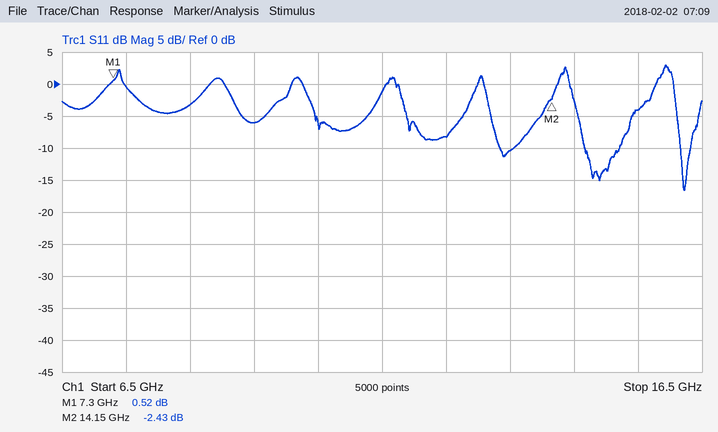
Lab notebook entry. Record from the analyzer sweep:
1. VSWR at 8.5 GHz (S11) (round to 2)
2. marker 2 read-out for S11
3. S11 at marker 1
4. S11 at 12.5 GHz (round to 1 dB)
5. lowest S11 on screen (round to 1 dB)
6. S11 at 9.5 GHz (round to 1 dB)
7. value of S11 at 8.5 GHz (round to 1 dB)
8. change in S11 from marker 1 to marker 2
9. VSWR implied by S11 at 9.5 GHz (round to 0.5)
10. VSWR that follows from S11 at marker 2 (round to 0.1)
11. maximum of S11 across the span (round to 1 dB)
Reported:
6
-2.43 dB
0.52 dB
-8 dB
-17 dB
-6 dB
-3 dB
-2.95 dB
3.0
7.2
3 dB
